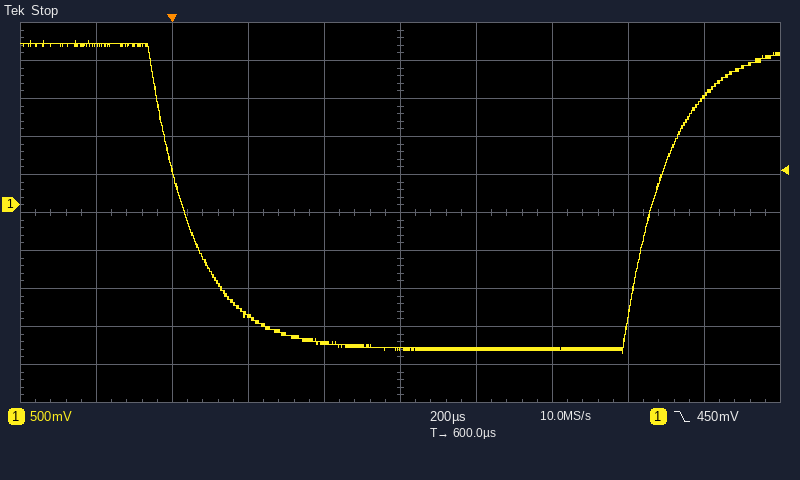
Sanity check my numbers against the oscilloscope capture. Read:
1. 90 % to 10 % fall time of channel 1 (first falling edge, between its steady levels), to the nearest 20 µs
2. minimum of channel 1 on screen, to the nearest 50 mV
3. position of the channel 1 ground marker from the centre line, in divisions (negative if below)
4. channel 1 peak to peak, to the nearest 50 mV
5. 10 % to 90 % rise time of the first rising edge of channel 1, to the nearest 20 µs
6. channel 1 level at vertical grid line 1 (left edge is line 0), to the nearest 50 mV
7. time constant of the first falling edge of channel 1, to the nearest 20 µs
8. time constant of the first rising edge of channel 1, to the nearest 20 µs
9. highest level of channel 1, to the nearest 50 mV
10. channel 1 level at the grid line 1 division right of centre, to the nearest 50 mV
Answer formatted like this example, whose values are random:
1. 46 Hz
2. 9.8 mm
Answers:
1. 260 µs
2. -1.95 V
3. +0.2 div
4. 4.10 V
5. 260 µs
6. 2.10 V
7. 120 µs
8. 120 µs
9. 2.15 V
10. -1.90 V
